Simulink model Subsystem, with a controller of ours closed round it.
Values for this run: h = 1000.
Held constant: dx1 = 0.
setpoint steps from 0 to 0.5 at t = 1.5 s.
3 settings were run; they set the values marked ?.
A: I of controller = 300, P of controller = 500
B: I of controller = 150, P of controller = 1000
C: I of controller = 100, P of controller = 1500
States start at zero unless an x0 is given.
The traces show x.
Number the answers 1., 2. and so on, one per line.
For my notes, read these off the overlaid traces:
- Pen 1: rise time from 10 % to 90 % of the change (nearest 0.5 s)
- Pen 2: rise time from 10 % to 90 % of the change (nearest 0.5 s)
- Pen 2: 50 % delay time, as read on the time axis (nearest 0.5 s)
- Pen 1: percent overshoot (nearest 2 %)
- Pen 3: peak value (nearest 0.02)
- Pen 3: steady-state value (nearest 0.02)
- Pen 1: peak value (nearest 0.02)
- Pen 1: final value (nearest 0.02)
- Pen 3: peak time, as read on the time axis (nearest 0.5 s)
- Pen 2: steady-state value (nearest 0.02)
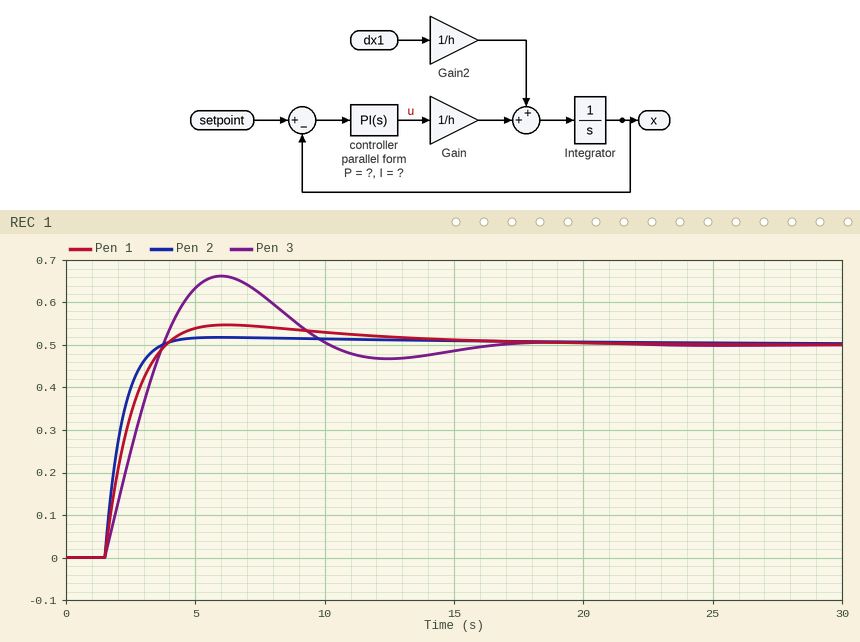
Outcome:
1. 1.5 s
2. 1.5 s
3. 2.0 s
4. 10 %
5. 0.66
6. 0.50
7. 0.54
8. 0.50
9. 6.0 s
10. 0.50
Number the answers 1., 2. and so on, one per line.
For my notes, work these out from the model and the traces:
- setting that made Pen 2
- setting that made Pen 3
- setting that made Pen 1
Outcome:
1. C
2. A
3. B
